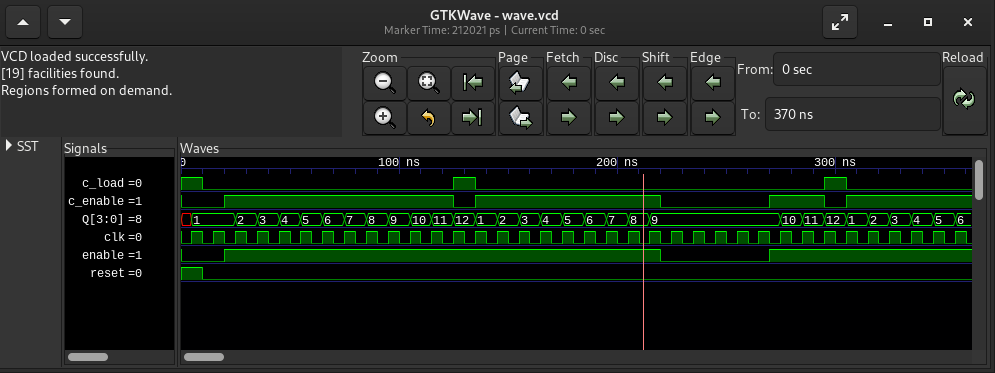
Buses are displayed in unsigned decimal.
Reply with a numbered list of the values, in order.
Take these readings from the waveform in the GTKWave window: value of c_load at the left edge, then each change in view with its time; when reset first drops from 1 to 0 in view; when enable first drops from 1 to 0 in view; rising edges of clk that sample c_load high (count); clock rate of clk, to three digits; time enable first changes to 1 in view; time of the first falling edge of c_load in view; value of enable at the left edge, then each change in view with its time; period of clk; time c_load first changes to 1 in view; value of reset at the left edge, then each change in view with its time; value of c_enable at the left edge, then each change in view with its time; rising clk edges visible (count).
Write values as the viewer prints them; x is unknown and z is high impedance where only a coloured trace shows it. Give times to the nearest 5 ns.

1. 1, 0 at 10 ns, 1 at 125 ns, 0 at 135 ns, 1 at 295 ns, 0 at 305 ns
2. 10 ns
3. 220 ns
4. 3
5. 100 MHz
6. 20 ns
7. 10 ns
8. 0, 1 at 20 ns, 0 at 220 ns, 1 at 270 ns
9. 10 ns
10. 125 ns
11. 1, 0 at 10 ns
12. 0, 1 at 20 ns, 0 at 125 ns, 1 at 135 ns, 0 at 220 ns, 1 at 270 ns, 0 at 295 ns, 1 at 305 ns
13. 36
